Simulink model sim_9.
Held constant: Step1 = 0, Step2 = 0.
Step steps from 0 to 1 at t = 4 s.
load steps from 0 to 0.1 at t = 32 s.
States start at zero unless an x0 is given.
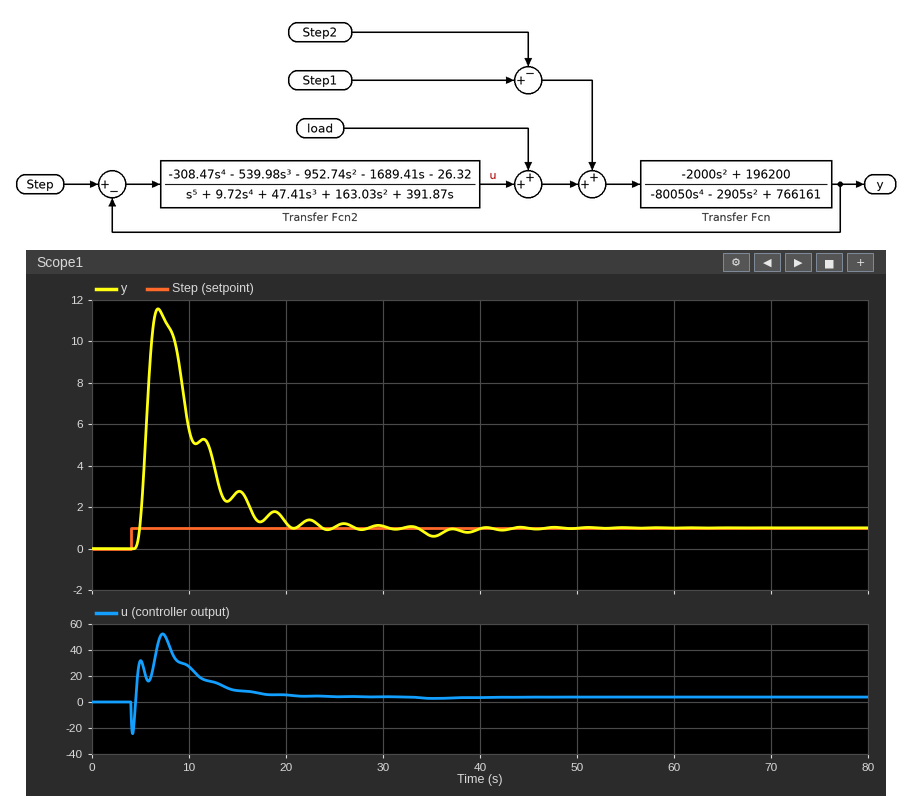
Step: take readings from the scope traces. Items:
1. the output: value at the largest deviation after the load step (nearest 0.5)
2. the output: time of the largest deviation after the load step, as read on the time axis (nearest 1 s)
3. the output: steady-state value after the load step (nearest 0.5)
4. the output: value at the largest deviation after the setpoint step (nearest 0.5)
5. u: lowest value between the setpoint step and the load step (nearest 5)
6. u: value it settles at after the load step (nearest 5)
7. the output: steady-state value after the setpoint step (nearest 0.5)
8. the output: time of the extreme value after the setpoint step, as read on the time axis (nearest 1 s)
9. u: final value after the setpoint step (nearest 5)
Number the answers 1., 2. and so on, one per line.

1. 0.5
2. 35 s
3. 1.0
4. 11.5
5. -25
6. 5
7. 1.0
8. 7 s
9. 5
